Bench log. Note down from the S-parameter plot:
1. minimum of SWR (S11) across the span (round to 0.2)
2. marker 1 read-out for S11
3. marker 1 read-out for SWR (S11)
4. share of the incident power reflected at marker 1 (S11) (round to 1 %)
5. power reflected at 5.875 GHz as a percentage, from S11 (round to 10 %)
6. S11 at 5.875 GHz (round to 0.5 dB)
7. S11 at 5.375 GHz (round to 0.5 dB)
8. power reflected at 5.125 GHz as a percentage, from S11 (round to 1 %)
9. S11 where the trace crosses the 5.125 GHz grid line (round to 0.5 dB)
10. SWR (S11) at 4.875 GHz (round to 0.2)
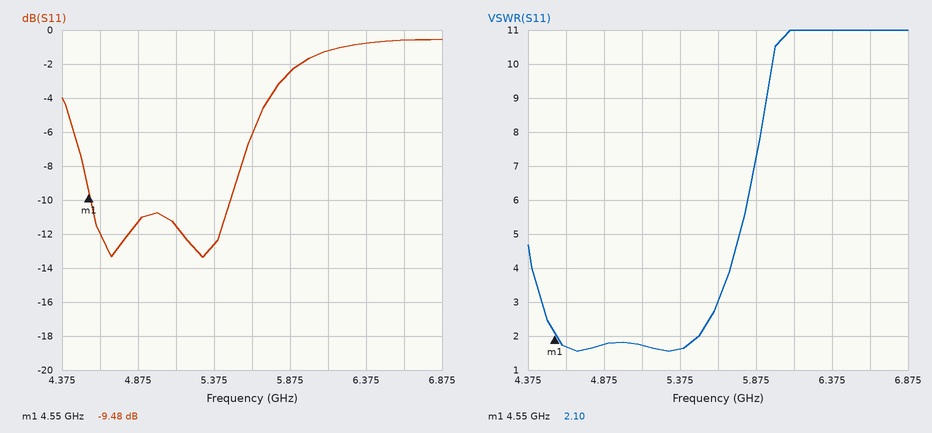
1.6
-9.48 dB
2.10
11 %
60 %
-2.5 dB
-12.5 dB
7 %
-11.5 dB
1.8
